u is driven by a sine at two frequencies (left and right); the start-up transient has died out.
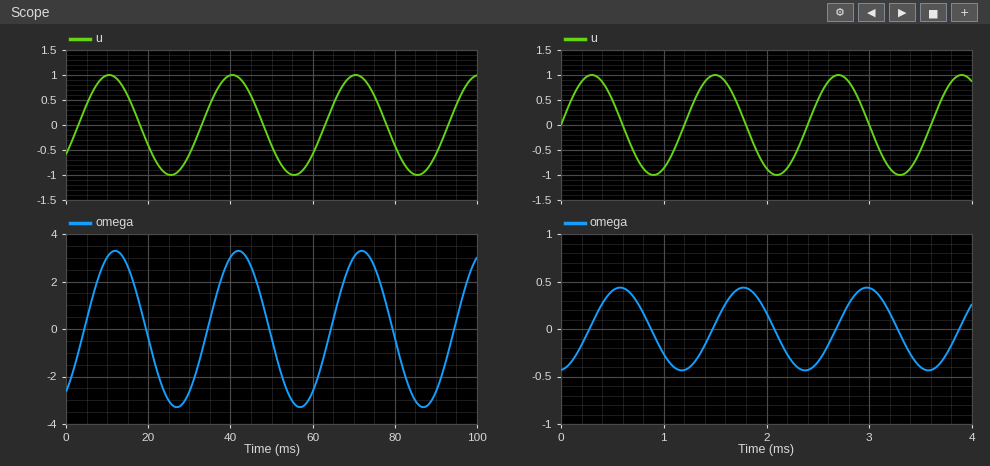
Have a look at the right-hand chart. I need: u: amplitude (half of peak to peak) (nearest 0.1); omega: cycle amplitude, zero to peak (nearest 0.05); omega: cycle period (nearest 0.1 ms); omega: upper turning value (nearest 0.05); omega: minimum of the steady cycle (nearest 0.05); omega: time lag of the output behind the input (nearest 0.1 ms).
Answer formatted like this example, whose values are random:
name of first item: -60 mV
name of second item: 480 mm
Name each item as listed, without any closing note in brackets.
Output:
u: amplitude (half of peak to peak): 1.0
omega: cycle amplitude, zero to peak: 0.45
omega: cycle period: 1.2 ms
omega: upper turning value: 0.45
omega: minimum of the steady cycle: -0.45
omega: time lag of the output behind the input: 0.3 ms
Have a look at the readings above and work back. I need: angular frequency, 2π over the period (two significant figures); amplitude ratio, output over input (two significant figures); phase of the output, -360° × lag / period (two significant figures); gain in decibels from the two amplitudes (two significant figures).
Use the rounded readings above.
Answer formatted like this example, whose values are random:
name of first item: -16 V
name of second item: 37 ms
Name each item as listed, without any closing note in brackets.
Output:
angular frequency, 2π over the period: 5.2 rad/ms
amplitude ratio, output over input: 0.45
phase of the output, -360° × lag / period: -90°
gain in decibels from the two amplitudes: -6.9 dB
